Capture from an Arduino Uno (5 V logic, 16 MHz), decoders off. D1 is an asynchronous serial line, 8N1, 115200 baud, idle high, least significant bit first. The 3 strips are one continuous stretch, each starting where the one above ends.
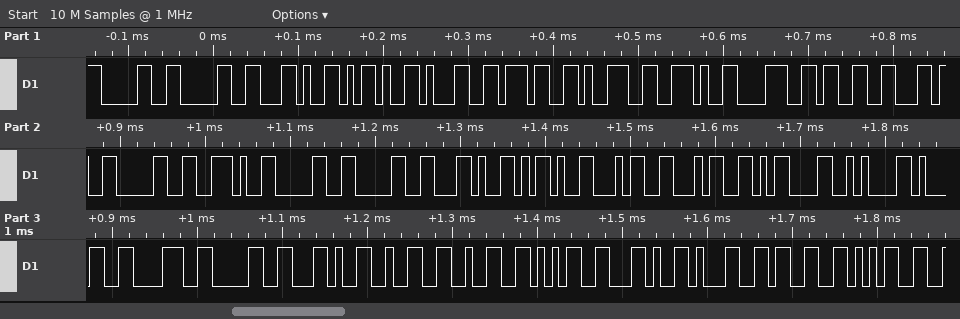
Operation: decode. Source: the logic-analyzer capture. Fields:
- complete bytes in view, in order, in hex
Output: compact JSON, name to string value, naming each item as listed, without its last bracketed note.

{"complete bytes in view, in order, in hex": "30 30 2C 2D 31 37 39 2E 38 33 2C 30 2E 30 30 2C 2D 34 34 0D 0A 31 38 30 2C 32 32 35 2C 31 33 35"}
